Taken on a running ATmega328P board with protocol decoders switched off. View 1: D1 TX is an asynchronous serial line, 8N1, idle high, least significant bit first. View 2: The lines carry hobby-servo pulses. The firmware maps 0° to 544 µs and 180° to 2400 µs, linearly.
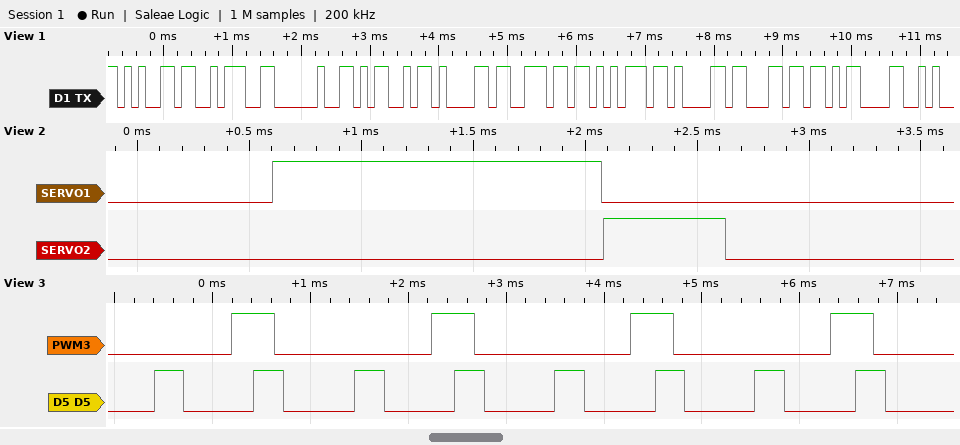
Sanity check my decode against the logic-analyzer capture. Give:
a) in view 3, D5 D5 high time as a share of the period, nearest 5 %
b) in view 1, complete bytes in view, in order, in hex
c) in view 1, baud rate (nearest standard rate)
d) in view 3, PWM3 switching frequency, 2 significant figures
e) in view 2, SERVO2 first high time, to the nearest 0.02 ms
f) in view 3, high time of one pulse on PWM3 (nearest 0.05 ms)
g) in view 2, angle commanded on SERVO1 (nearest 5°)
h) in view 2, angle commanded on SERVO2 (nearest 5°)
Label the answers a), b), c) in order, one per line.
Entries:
a) 30 %
b) 65 3A 20 4D 61 6E 75 61 6C 0D
c) 9600 baud
d) 490 Hz
e) 0.54 ms
f) 0.45 ms
g) 90°
h) 0°
